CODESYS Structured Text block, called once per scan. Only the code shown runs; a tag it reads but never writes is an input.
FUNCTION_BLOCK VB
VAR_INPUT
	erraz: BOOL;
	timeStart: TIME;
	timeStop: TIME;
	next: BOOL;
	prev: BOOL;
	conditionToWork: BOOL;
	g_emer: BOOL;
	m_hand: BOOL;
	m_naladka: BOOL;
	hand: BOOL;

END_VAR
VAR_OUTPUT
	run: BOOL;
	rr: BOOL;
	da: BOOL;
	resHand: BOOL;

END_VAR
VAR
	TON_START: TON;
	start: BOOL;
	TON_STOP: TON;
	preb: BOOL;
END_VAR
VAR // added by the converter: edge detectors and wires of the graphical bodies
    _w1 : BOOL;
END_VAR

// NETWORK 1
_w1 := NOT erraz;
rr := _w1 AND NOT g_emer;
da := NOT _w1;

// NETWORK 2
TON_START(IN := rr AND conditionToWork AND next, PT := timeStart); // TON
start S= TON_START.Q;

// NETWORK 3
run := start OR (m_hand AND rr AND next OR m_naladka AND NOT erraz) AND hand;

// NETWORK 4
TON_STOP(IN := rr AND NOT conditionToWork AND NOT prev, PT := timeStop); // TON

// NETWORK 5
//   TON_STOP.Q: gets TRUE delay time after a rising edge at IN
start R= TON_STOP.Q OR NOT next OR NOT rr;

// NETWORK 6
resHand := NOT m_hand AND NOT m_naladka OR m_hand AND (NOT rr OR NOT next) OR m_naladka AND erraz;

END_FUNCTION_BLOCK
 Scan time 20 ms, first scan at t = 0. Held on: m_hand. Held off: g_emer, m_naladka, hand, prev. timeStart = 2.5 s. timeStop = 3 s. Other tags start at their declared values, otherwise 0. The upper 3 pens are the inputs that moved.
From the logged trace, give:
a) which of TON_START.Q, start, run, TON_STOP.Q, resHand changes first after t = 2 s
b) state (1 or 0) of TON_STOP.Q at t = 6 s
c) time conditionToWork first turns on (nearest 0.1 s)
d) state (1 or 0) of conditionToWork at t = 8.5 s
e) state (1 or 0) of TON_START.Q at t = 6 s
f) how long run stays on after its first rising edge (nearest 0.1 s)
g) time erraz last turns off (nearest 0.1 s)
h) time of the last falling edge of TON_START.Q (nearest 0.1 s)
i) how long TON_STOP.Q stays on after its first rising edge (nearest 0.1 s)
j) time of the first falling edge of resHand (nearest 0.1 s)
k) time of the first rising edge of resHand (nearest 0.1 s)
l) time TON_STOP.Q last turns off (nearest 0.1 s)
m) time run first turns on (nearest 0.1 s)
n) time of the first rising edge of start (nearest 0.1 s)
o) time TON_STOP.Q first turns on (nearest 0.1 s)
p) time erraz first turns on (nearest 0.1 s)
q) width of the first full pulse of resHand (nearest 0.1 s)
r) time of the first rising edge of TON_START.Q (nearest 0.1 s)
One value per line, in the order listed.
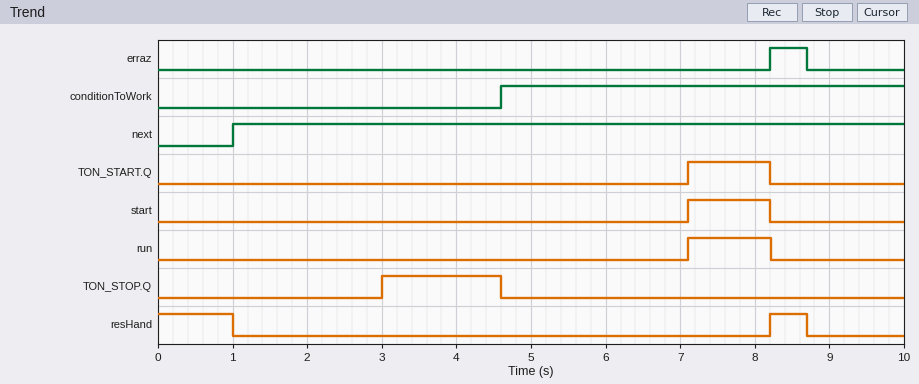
TON_STOP.Q
0
4.6 s
1
0
1.1 s
8.7 s
8.2 s
1.6 s
1.0 s
8.2 s
4.6 s
7.1 s
7.1 s
3.0 s
8.2 s
0.5 s
7.1 s
